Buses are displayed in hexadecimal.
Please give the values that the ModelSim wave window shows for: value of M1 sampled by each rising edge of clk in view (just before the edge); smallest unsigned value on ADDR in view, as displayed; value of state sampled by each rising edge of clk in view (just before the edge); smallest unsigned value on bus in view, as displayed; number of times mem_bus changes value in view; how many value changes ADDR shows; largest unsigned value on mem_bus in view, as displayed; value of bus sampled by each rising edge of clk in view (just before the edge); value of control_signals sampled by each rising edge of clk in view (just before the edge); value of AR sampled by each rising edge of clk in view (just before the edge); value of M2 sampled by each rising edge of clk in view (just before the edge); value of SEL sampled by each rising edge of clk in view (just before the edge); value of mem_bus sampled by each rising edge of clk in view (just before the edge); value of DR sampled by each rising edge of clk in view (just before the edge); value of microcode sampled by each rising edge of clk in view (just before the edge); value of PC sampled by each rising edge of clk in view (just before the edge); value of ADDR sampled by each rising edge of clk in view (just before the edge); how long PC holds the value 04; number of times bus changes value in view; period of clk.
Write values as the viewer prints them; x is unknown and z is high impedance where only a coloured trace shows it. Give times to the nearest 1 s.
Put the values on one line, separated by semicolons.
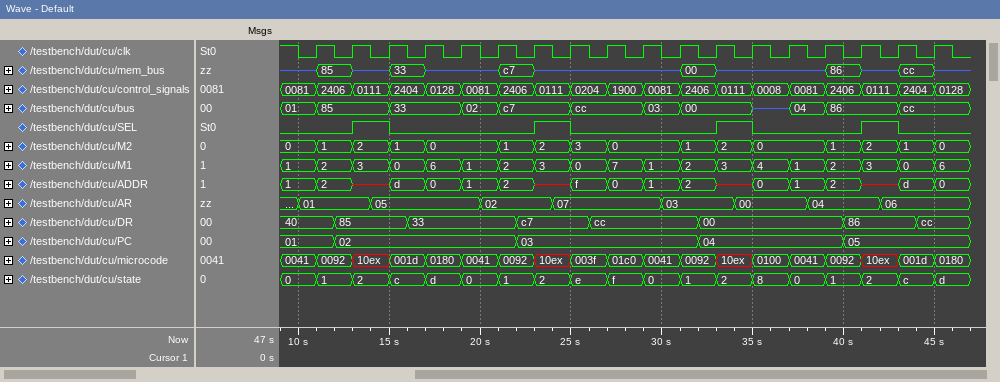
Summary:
1, 2, 3, 0, 6, 1, 2, 3, 0, 7, 1, 2, 3, 4, 1, 2, 3, 0; 0; 0, 1, 2, c, d, 0, 1, 2, e, f, 0, 1, 2, 8, 0, 1, 2, c; 00; 12; 18; cc; 01, 85, 85, 33, 33, 02, c7, c7, cc, cc, 03, 00, 00, z, 04, 86, 86, cc; 0081, 2406, 0111, 2404, 0128, 0081, 2406, 0111, 0204, 1900, 0081, 2406, 0111, 0008, 0081, 2406, 0111, 2404; 01, 01, 05, 05, 05, 02, 02, 07, 07, 07, 03, 03, 00, 00, 04, 04, 06, 06; 0, 1, 2, 1, 0, 0, 1, 2, 3, 0, 0, 1, 2, 0, 0, 1, 2, 1; 0 0 1 0 0 0 0 1 0 0 0 0 1 0 0 0 1 0; z, 85, z, 33, z, z, c7, z, z, z, z, 00, z, z, z, 86, z, cc; 40, 85, 85, 33, 33, 33, c7, c7, cc, cc, cc, 00, 00, 00, 00, 86, 86, cc; 0041, 0092, 10ex, 001d, 0180, 0041, 0092, 10ex, 003f, 01c0, 0041, 0092, 10ex, 0100, 0041, 0092, 10ex, 001d; 01, 02, 02, 02, 02, 02, 03, 03, 03, 03, 03, 04, 04, 04, 04, 05, 05, 05; 1, 2, x, d, 0, 1, 2, x, f, 0, 1, 2, x, 0, 1, 2, x, d; 8 s; 11; 2 s
